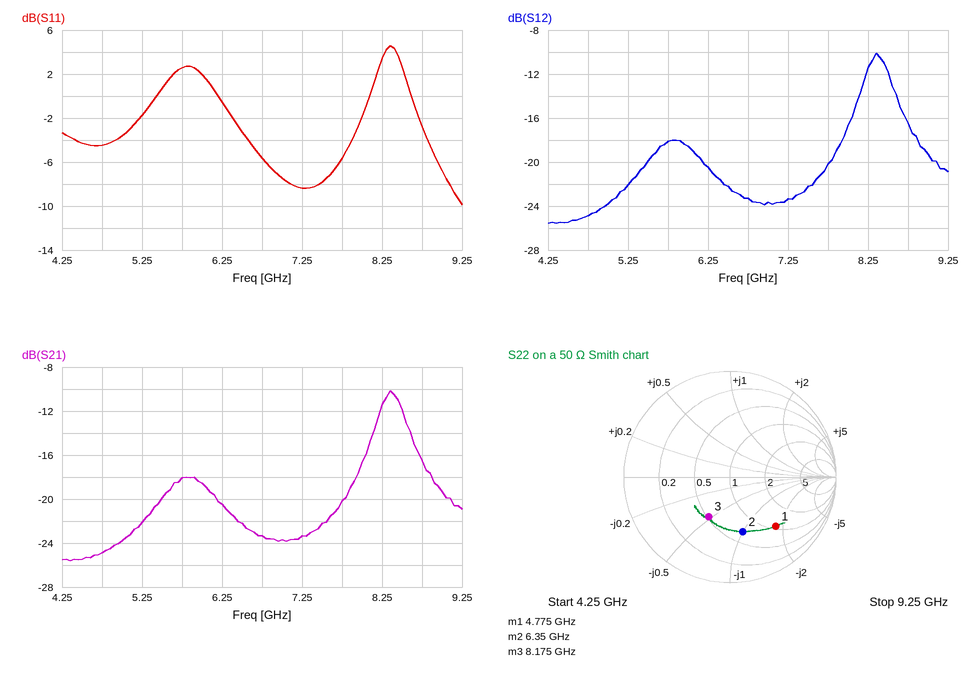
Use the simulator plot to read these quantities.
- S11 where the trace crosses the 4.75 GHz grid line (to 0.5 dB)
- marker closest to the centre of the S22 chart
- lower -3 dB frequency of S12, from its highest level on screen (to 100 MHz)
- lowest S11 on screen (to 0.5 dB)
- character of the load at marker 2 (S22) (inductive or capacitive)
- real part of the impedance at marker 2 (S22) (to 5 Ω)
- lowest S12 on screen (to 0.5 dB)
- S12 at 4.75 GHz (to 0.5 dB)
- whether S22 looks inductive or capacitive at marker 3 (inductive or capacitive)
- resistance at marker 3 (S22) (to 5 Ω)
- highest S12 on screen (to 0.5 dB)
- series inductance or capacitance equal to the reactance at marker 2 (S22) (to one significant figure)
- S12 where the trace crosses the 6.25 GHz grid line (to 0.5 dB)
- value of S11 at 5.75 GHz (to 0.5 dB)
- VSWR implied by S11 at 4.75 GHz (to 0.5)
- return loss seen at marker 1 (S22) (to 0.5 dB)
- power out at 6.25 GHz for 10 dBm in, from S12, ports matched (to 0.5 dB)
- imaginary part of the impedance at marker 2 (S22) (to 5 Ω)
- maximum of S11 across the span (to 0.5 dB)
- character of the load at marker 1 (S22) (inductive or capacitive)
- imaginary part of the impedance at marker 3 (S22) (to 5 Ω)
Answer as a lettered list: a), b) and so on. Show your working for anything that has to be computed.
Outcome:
a) -4.5 dB
b) marker 3
c) 8.2 GHz
d) -10.0 dB
e) capacitive
f) 35 Ω
g) -25.5 dB
h) -25.0 dB
i) capacitive
j) 25 Ω
k) -10.0 dB
l) C = 1/(2π × 6.35 GHz × 50 Ω) ≈ 501 fF, so 500 fF to one significant figure
m) -20.5 dB
n) 2.5 dB
o) |Γ| = 10^(-4.5/20) = 0.5957; VSWR = (1 + 0.5957)/(1 − 0.5957) ≈ 4.0
p) 4.0 dB
q) 10 dBm + (-20.5 dB) = -10.5 dBm
r) -50 Ω
s) 4.5 dB
t) capacitive
u) -25 Ω
